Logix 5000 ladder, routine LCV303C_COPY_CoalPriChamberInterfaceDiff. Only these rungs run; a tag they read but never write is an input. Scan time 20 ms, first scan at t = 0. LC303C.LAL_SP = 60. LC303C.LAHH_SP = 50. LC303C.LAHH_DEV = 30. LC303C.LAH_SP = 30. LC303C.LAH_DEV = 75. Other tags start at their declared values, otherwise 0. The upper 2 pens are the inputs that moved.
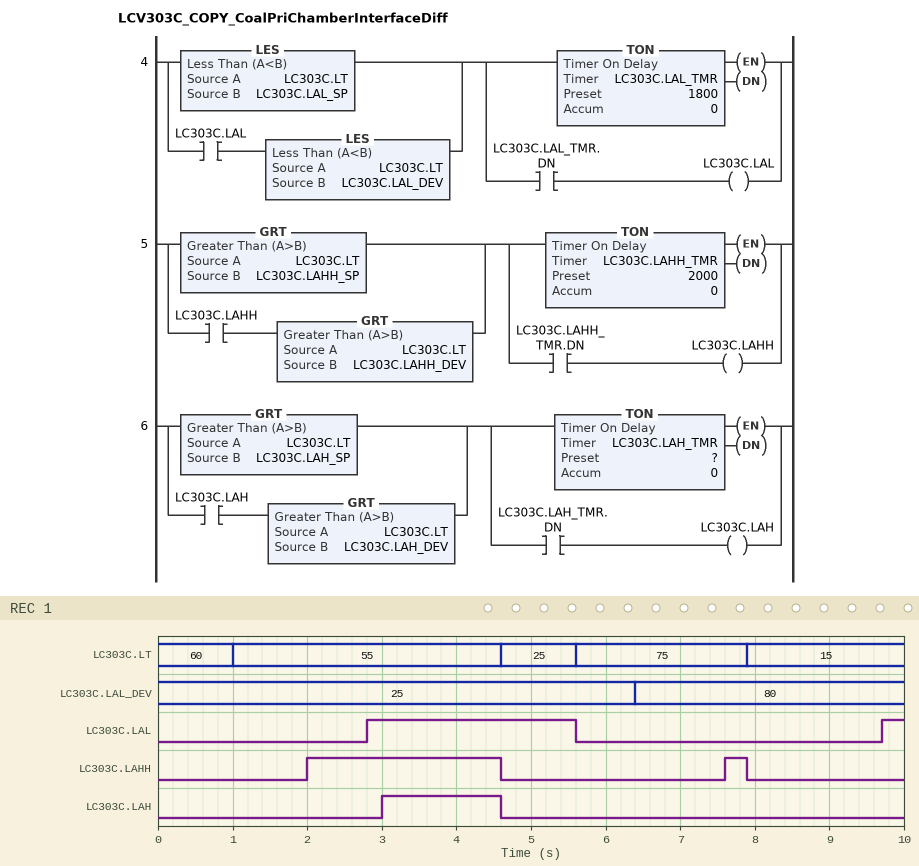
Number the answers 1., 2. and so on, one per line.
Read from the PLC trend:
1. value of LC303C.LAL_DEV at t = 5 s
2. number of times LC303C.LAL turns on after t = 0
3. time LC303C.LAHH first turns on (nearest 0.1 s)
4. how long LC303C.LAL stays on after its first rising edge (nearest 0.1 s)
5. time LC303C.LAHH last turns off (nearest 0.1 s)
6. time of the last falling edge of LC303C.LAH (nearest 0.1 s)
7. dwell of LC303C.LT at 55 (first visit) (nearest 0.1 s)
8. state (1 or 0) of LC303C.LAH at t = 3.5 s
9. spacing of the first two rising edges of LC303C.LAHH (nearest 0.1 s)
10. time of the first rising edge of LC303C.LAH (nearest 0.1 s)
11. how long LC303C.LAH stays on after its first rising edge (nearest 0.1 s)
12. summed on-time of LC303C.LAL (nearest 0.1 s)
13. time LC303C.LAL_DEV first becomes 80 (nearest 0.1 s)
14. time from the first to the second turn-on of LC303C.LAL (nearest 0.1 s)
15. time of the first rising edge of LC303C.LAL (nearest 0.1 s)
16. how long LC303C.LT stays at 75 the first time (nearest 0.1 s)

1. 25
2. 2
3. 2.0 s
4. 2.8 s
5. 7.9 s
6. 4.6 s
7. 3.6 s
8. 1
9. 5.6 s
10. 3.0 s
11. 1.6 s
12. 3.1 s
13. 6.4 s
14. 6.9 s
15. 2.8 s
16. 2.3 s
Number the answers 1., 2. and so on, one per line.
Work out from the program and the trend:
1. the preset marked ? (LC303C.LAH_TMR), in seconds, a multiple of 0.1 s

1. 3.0 s
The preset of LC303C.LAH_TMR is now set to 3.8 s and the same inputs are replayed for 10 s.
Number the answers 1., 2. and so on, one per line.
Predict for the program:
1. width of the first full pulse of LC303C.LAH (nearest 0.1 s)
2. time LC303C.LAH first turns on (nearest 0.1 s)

1. 0.8 s
2. 3.8 s
